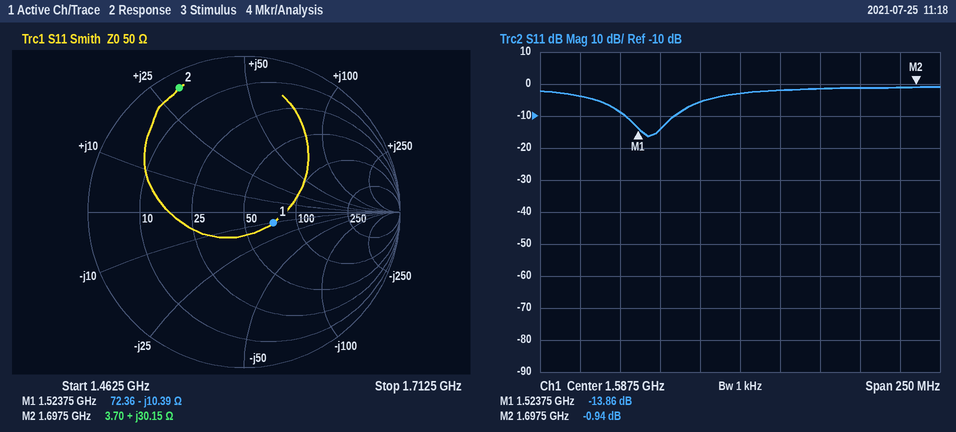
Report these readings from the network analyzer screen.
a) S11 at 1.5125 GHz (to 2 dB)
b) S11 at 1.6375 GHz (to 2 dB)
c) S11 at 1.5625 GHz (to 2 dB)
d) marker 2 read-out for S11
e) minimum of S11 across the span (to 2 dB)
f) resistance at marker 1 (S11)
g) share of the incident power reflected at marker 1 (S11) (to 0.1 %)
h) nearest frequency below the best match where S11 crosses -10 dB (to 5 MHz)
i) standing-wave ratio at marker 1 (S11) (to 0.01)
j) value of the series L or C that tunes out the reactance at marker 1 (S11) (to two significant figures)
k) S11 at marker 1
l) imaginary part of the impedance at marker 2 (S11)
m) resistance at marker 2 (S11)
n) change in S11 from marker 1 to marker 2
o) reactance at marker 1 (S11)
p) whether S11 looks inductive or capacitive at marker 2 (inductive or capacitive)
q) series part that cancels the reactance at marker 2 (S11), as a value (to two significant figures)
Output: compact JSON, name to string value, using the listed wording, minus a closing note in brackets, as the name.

{"S11 at 1.5125 GHz": "-8 dB", "S11 at 1.6375 GHz": "-2 dB", "S11 at 1.5625 GHz": "-6 dB", "marker 2 read-out for S11": "-0.94 dB", "minimum of S11 across the span": "-16 dB", "resistance at marker 1": "72.36 Ω", "share of the incident power reflected at marker 1 (S11)": "4.1 %", "nearest frequency below the best match where S11 crosses -10 dB": "1.515 GHz", "standing-wave ratio at marker 1 (S11)": "1.50", "value of the series L or C that tunes out the reactance at marker 1 (S11)": "1.1 nH", "S11 at marker 1": "-13.86 dB", "imaginary part of the impedance at marker 2": "+30.15 Ω", "resistance at marker 2": "3.70 Ω", "change in S11 from marker 1 to marker 2": "12.92 dB", "reactance at marker 1": "-10.39 Ω", "whether S11 looks inductive or capacitive at marker 2": "inductive", "series part that cancels the reactance at marker 2 (S11), as a value": "3.1 pF"}
